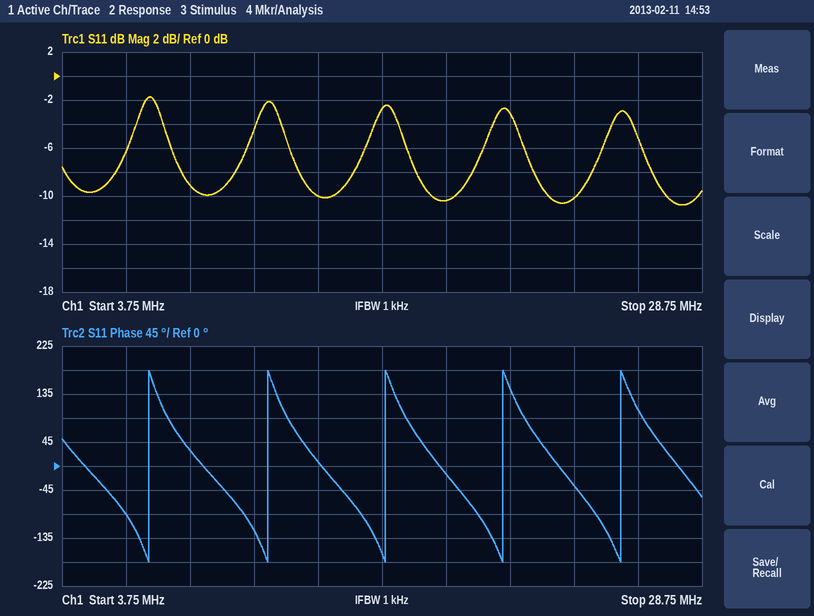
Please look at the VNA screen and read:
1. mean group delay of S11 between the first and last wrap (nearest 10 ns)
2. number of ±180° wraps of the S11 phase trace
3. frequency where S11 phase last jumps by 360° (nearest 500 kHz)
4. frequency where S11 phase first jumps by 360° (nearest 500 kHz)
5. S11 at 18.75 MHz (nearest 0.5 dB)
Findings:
220 ns
5
25.5 MHz
7.0 MHz
-10.5 dB
